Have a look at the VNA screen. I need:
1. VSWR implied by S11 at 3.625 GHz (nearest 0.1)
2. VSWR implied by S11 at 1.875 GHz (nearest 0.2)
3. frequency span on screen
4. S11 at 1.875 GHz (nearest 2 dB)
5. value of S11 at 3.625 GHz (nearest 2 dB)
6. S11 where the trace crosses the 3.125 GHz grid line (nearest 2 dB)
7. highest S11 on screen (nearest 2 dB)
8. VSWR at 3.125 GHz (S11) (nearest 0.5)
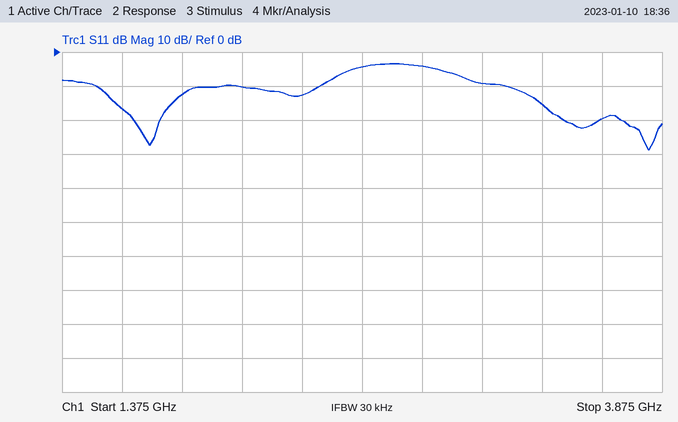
1.2
1.6
2.5 GHz
-12 dB
-20 dB
-10 dB
-4 dB
2.0
